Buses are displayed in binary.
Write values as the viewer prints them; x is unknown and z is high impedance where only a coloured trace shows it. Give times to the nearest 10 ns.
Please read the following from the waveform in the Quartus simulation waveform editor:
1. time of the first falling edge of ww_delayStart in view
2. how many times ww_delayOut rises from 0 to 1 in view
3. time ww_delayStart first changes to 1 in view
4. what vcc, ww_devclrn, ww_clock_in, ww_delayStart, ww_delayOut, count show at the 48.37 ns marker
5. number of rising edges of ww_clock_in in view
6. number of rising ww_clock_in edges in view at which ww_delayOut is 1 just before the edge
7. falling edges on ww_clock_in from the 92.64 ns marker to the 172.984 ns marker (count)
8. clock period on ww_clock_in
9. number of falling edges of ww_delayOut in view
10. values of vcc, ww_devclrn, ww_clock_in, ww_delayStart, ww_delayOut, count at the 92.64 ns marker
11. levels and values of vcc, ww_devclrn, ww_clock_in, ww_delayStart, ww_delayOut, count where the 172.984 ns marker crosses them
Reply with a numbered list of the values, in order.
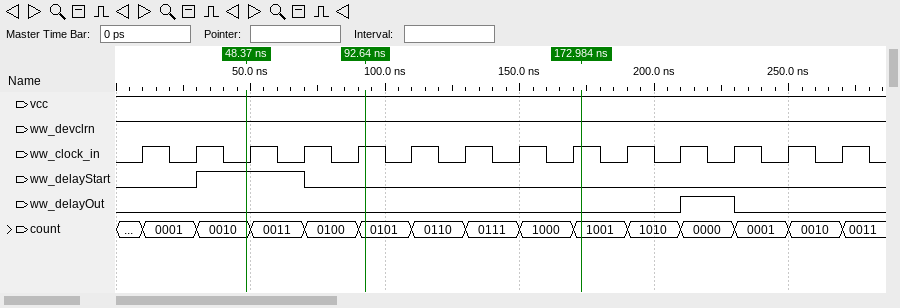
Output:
1. 70 ns
2. 1
3. 30 ns
4. vcc=1, ww_devclrn=1, ww_clock_in=0, ww_delayStart=1, ww_delayOut=0, count=0010
5. 14
6. 1
7. 4
8. 20 ns
9. 1
10. vcc=1, ww_devclrn=1, ww_clock_in=1, ww_delayStart=0, ww_delayOut=0, count=0101
11. vcc=1, ww_devclrn=1, ww_clock_in=1, ww_delayStart=0, ww_delayOut=0, count=1001
